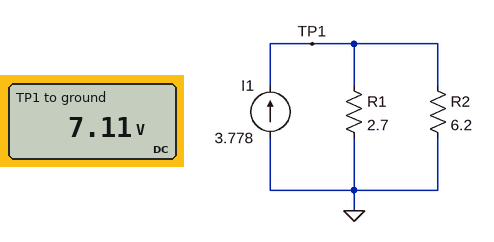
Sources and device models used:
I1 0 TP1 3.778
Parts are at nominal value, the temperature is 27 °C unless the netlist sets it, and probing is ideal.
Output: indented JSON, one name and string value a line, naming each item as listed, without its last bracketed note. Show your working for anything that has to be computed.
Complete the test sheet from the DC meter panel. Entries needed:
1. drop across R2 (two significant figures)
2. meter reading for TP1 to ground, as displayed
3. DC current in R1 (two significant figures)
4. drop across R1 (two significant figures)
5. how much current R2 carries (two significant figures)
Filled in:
{
  "drop across R2": "7.11 V = 7.1 V",
  "meter reading for TP1 to ground, as displayed": "7.11 V",
  "DC current in R1": "(7.11 V) / 2.7 Ω = 2.6 A",
  "drop across R1": "7.11 V = 7.1 V",
  "how much current R2 carries": "(7.11 V) / 6.2 Ω = 1.1 A"
}
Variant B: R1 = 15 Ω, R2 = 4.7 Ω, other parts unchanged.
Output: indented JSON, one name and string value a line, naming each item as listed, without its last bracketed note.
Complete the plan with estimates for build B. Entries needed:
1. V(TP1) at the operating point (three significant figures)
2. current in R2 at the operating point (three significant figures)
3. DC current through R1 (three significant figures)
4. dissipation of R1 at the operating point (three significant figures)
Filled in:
{
  "V(TP1) at the operating point": "13.5 V",
  "current in R2 at the operating point": "2.88 A",
  "DC current through R1": "901 mA",
  "dissipation of R1 at the operating point": "12.2 W"
}
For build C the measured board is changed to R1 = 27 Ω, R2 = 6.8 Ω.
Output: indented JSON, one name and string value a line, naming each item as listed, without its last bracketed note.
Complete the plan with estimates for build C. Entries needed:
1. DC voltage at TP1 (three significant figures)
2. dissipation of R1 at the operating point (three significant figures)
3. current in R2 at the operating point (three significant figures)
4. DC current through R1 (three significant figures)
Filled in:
{
  "DC voltage at TP1": "20.5 V",
  "dissipation of R1 at the operating point": "15.6 W",
  "current in R2 at the operating point": "3.02 A",
  "DC current through R1": "760 mA"
}
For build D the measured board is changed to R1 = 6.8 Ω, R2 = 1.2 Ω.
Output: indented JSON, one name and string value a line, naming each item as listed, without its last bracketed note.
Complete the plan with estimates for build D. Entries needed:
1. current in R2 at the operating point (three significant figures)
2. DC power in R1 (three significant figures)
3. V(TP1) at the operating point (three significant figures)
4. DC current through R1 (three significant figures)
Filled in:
{
  "current in R2 at the operating point": "3.21 A",
  "DC power in R1": "2.18 W",
  "V(TP1) at the operating point": "3.85 V",
  "DC current through R1": "567 mA"
}
